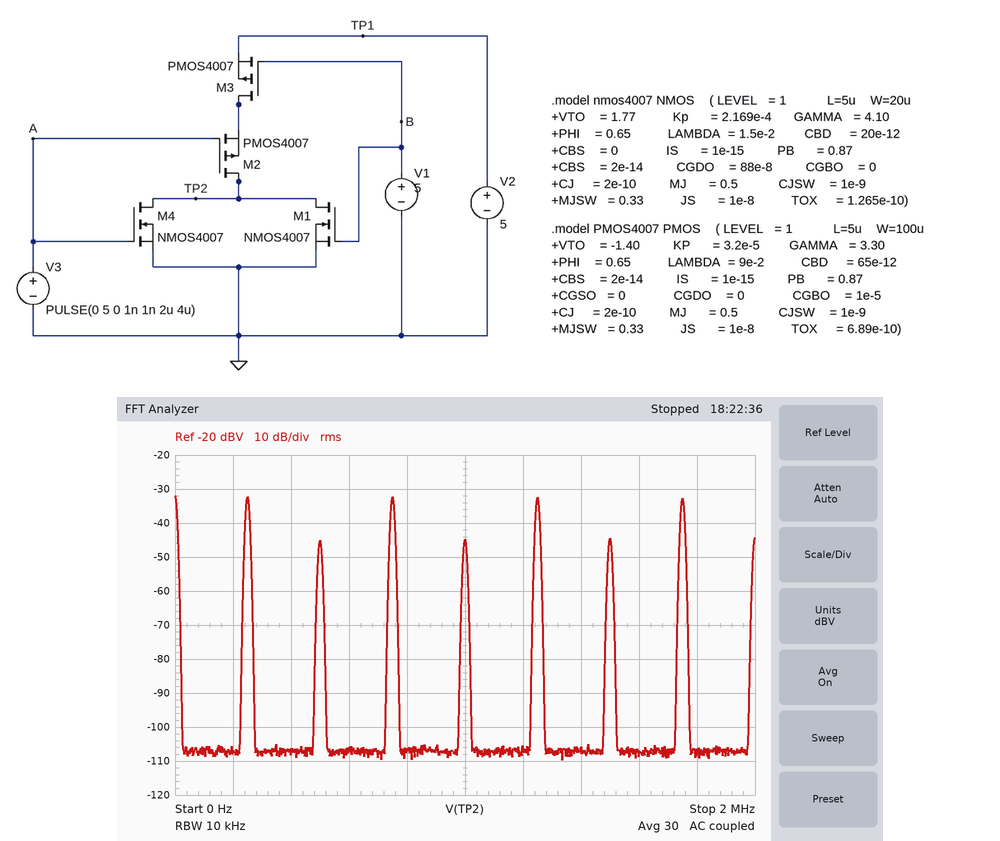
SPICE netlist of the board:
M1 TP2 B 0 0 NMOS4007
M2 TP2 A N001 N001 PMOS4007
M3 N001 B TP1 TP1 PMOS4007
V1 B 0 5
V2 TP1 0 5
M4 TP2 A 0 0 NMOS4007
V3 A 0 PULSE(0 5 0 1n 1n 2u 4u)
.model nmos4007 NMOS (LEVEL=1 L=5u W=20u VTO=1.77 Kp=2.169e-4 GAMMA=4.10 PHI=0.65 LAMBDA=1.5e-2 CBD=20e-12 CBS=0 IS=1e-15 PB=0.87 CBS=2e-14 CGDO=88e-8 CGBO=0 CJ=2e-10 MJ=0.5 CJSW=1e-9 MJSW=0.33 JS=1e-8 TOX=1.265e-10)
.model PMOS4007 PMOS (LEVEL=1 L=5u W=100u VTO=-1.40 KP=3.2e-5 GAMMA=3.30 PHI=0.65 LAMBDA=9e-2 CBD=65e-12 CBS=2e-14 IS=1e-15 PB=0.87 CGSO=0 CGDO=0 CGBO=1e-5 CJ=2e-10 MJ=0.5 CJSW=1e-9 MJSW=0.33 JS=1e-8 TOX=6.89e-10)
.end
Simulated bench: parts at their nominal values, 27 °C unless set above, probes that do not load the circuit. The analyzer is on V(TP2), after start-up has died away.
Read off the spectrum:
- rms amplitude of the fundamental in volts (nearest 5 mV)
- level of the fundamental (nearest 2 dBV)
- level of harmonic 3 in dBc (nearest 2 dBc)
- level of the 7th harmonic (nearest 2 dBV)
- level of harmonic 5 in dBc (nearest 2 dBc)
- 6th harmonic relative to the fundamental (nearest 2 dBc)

25 mV
-32 dBV
0 dBc
-32 dBV
0 dBc
-12 dBc
